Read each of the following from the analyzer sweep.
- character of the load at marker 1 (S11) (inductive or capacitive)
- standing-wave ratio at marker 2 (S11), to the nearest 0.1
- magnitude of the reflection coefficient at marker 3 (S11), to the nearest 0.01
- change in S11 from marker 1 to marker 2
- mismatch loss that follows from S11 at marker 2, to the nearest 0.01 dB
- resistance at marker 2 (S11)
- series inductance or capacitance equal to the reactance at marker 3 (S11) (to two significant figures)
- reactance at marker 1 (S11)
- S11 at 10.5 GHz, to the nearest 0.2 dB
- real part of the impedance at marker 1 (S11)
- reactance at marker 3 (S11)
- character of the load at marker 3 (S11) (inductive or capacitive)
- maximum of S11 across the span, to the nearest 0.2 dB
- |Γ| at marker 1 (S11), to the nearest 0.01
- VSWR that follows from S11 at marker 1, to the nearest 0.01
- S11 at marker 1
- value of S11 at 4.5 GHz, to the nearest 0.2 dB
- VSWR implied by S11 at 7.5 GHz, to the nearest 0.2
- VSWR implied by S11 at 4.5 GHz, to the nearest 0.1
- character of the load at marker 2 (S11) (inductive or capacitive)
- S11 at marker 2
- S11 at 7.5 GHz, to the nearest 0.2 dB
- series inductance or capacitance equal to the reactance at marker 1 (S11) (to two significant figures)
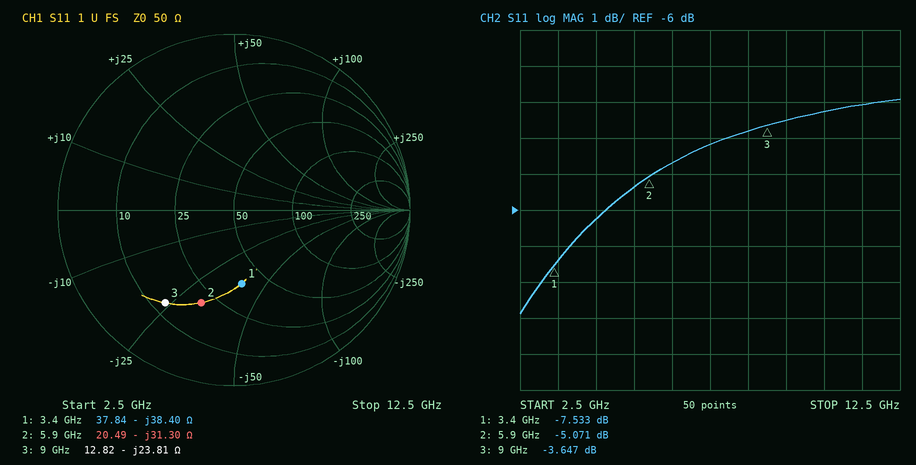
capacitive
3.5
0.66
2.462 dB
1.62 dB
20.49 Ω
740 fF
-38.40 Ω
-3.2 dB
37.84 Ω
-23.81 Ω
capacitive
-3.0 dB
0.42
2.45
-7.533 dB
-6.2 dB
4.2
2.9
capacitive
-5.071 dB
-4.2 dB
1.2 pF
